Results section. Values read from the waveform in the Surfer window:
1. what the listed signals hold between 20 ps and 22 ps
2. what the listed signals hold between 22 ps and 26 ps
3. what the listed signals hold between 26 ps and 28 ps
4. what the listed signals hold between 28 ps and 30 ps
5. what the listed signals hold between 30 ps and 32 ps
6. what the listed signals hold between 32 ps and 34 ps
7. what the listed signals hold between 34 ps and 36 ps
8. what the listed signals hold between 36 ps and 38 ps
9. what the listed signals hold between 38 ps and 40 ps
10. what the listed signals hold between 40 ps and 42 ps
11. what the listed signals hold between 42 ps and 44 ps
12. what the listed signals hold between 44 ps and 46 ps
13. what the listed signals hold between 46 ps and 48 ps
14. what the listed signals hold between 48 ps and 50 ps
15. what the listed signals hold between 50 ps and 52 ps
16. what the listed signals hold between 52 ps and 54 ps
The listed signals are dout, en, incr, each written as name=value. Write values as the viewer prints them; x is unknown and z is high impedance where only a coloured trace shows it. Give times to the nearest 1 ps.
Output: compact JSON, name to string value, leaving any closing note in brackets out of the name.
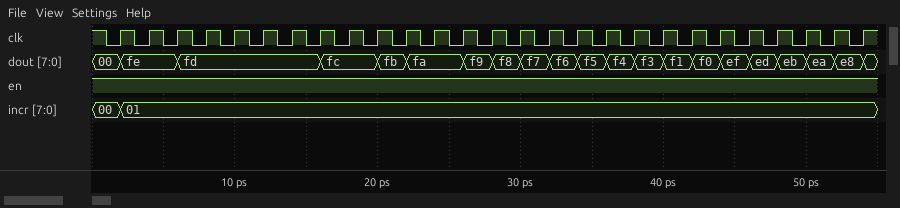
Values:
{"what the listed signals hold between 20 ps and 22 ps": "dout=fb, en=1, incr=01", "what the listed signals hold between 22 ps and 26 ps": "dout=fa, en=1, incr=01", "what the listed signals hold between 26 ps and 28 ps": "dout=f9, en=1, incr=01", "what the listed signals hold between 28 ps and 30 ps": "dout=f8, en=1, incr=01", "what the listed signals hold between 30 ps and 32 ps": "dout=f7, en=1, incr=01", "what the listed signals hold between 32 ps and 34 ps": "dout=f6, en=1, incr=01", "what the listed signals hold between 34 ps and 36 ps": "dout=f5, en=1, incr=01", "what the listed signals hold between 36 ps and 38 ps": "dout=f4, en=1, incr=01", "what the listed signals hold between 38 ps and 40 ps": "dout=f3, en=1, incr=01", "what the listed signals hold between 40 ps and 42 ps": "dout=f1, en=1, incr=01", "what the listed signals hold between 42 ps and 44 ps": "dout=f0, en=1, incr=01", "what the listed signals hold between 44 ps and 46 ps": "dout=ef, en=1, incr=01", "what the listed signals hold between 46 ps and 48 ps": "dout=ed, en=1, incr=01", "what the listed signals hold between 48 ps and 50 ps": "dout=eb, en=1, incr=01", "what the listed signals hold between 50 ps and 52 ps": "dout=ea, en=1, incr=01", "what the listed signals hold between 52 ps and 54 ps": "dout=e8, en=1, incr=01"}
